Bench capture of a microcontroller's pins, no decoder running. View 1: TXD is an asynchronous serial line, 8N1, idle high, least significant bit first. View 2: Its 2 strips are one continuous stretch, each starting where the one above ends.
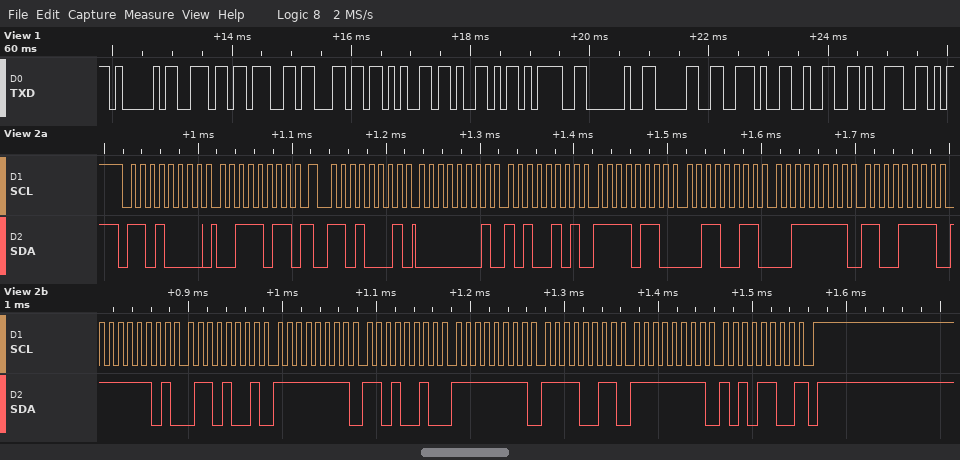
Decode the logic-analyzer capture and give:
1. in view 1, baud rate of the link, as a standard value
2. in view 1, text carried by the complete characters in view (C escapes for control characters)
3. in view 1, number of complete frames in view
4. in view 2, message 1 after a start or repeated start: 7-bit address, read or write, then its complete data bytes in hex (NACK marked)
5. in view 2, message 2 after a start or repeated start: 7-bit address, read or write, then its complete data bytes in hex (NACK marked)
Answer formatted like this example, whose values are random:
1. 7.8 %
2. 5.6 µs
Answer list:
1. 9600 baud
2. "AngleY= 0.29"
3. 12
4. 0x68 write: 3B
5. 0x68 read: 01 A5 F6 33 3F CF FD 69 FF D2 FF F3 FF AC NACK
